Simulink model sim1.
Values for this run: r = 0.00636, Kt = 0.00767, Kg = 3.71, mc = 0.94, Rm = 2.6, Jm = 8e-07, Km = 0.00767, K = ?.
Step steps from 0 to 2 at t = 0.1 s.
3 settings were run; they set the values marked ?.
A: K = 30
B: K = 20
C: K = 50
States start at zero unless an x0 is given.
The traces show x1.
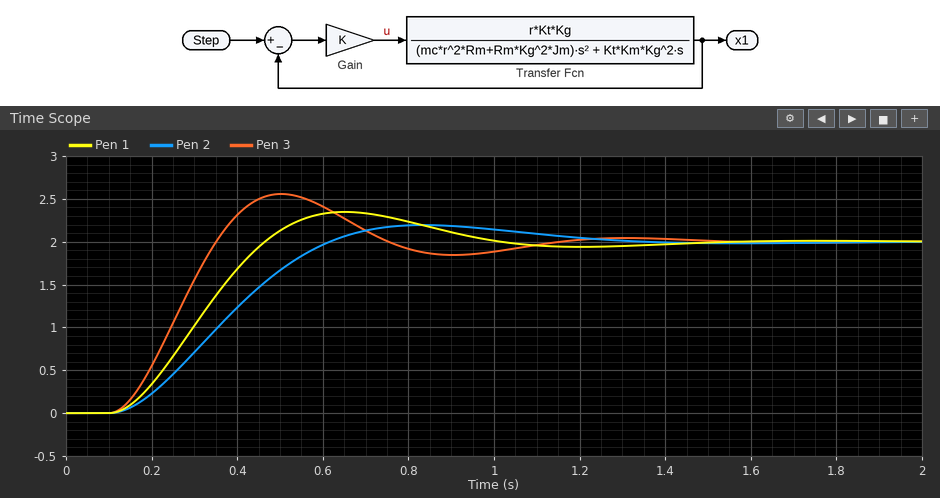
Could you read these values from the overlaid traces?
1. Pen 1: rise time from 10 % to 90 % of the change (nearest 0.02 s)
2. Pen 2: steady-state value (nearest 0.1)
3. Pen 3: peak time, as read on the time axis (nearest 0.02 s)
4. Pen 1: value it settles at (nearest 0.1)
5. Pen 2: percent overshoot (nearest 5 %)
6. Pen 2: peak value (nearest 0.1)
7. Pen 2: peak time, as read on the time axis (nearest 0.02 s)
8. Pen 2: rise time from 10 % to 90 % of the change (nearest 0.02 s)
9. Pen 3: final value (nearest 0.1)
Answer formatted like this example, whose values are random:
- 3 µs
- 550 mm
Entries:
- 0.24 s
- 2.0
- 0.50 s
- 2.0
- 10 %
- 2.2
- 0.84 s
- 0.34 s
- 2.0
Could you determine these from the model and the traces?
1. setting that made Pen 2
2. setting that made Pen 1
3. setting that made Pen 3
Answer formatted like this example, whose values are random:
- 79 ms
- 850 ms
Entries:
- B
- A
- C
